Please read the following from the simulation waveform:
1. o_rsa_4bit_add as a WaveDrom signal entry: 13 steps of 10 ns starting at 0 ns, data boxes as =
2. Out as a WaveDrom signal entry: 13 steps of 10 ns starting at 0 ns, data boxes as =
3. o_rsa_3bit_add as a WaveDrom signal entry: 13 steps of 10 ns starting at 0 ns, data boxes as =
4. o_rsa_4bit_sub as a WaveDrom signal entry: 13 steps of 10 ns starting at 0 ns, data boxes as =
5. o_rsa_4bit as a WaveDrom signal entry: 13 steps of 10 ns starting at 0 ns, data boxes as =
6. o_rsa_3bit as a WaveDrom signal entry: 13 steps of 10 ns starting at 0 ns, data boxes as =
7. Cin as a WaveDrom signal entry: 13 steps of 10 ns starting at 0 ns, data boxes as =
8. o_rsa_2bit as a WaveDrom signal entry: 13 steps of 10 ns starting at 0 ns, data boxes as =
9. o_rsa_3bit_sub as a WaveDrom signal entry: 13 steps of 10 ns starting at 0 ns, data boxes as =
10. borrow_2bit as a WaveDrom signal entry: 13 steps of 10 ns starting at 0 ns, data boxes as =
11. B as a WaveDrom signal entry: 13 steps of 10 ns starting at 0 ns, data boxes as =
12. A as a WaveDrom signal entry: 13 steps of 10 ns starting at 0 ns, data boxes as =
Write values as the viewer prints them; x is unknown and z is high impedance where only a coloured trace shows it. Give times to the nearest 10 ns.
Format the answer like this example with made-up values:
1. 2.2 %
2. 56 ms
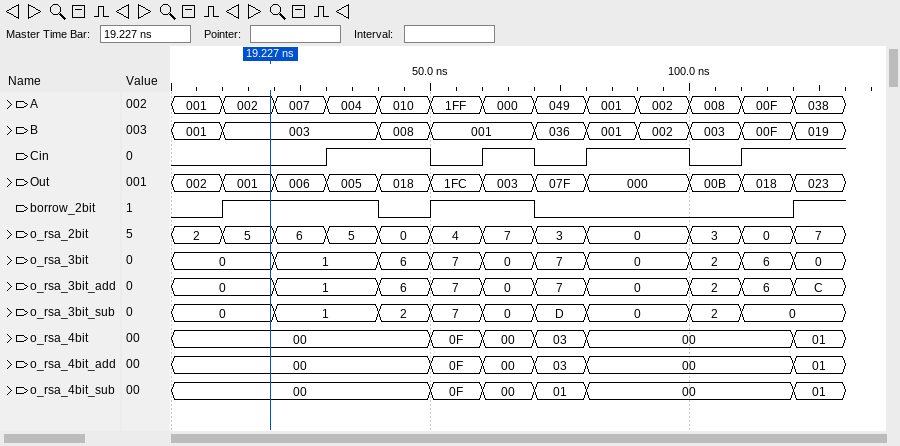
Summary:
1. {name: 'o_rsa_4bit_add', wave: '=....====...=', data: '00 0F 00 03 00 01'}
2. {name: 'Out', wave: '=========.===', data: '002 001 006 005 018 1FC 003 07F 000 00B 018 023'}
3. {name: 'o_rsa_3bit_add', wave: '=.=.=====.===', data: '0 1 6 7 0 7 0 2 6 C'}
4. {name: 'o_rsa_4bit_sub', wave: '=....====...=', data: '00 0F 00 01 00 01'}
5. {name: 'o_rsa_4bit', wave: '=....====...=', data: '00 0F 00 03 00 01'}
6. {name: 'o_rsa_3bit', wave: '=.=.=====.===', data: '0 1 6 7 0 7 0 2 6 0'}
7. {name: 'Cin', wave: '0..1.0101.01.'}
8. {name: 'o_rsa_2bit', wave: '=========.===', data: '2 5 6 5 0 4 7 3 0 3 0 7'}
9. {name: 'o_rsa_3bit_sub', wave: '=.=.=====.==.', data: '0 1 2 7 0 D 0 2 0'}
10. {name: 'borrow_2bit', wave: '01..01.0....1'}
11. {name: 'B', wave: '==..==.======', data: '001 003 008 001 036 001 002 003 00F 019'}
12. {name: 'A', wave: '=============', data: '001 002 007 004 010 1FF 000 049 001 002 008 00F 038'}
